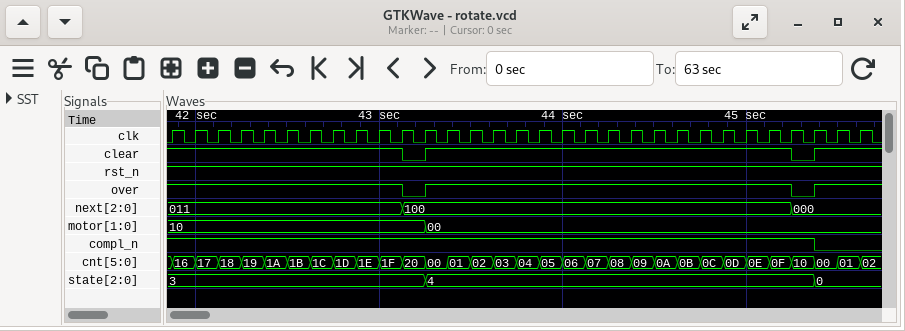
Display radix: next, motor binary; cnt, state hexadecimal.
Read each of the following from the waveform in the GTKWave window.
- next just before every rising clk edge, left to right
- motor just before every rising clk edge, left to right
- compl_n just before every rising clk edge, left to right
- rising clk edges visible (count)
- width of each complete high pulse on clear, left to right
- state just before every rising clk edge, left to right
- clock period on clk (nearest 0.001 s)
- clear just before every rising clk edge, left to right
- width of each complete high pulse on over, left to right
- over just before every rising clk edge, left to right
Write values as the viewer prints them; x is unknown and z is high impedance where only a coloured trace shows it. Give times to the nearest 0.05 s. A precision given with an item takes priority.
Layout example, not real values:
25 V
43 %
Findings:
011, 011, 011, 011, 011, 011, 011, 011, 011, 011, 011, 100, 100, 100, 100, 100, 100, 100, 100, 100, 100, 100, 100, 100, 100, 100, 100, 100, 000, 000, 000
10, 10, 10, 10, 10, 10, 10, 10, 10, 10, 10, 10, 00, 00, 00, 00, 00, 00, 00, 00, 00, 00, 00, 00, 00, 00, 00, 00, 00, 00, 00
1 1 1 1 1 1 1 1 1 1 1 1 1 1 1 1 1 1 1 1 1 1 1 1 1 1 1 1 1 0 0
31
2 s
3, 3, 3, 3, 3, 3, 3, 3, 3, 3, 3, 3, 4, 4, 4, 4, 4, 4, 4, 4, 4, 4, 4, 4, 4, 4, 4, 4, 4, 0, 0
0.125 s
1 1 1 1 1 1 1 1 1 1 1 0 1 1 1 1 1 1 1 1 1 1 1 1 1 1 1 1 0 1 1
2 s
1 1 1 1 1 1 1 1 1 1 1 0 1 1 1 1 1 1 1 1 1 1 1 1 1 1 1 1 0 1 1
